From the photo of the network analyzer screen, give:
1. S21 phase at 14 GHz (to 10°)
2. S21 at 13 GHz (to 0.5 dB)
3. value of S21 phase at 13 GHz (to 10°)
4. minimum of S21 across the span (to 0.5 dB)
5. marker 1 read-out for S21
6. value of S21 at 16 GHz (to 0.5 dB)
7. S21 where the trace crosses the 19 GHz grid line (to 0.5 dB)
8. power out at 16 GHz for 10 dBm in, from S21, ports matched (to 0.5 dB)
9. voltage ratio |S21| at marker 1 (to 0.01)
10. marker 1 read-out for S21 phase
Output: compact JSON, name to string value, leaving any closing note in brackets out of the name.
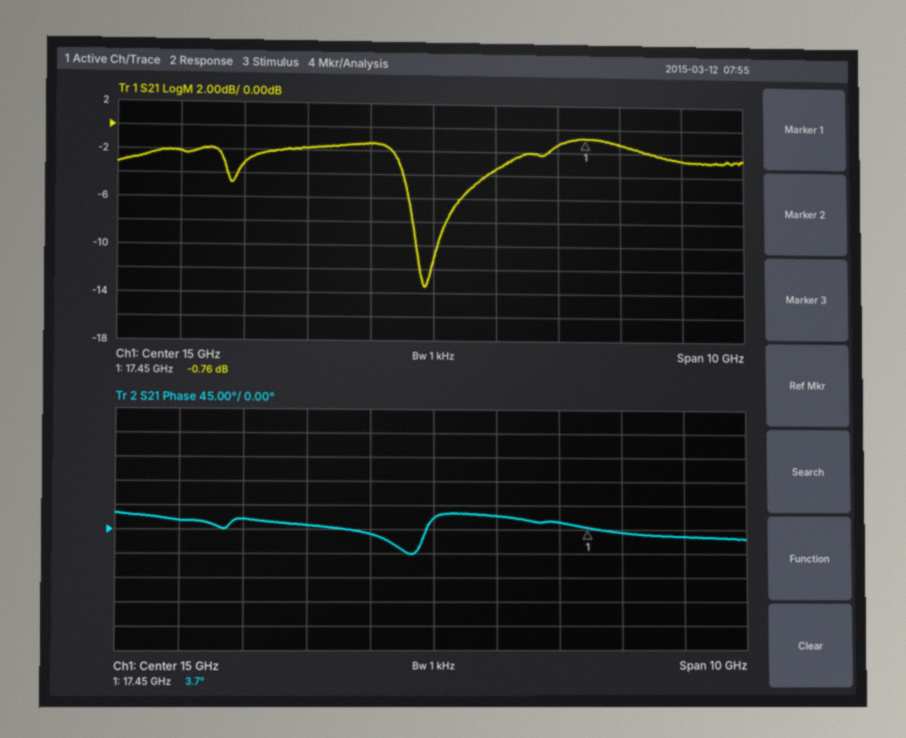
{"S21 phase at 14 GHz": "-10°", "S21 at 13 GHz": "-2.0 dB", "value of S21 phase at 13 GHz": "10°", "minimum of S21 across the span": "-13.5 dB", "marker 1 read-out for S21": "-0.76 dB", "value of S21 at 16 GHz": "-3.5 dB", "S21 where the trace crosses the 19 GHz grid line": "-2.5 dB", "power out at 16 GHz for 10 dBm in, from S21, ports matched": "6.5 dBm", "voltage ratio |S21| at marker 1": "0.92", "marker 1 read-out for S21 phase": "3.7°"}
